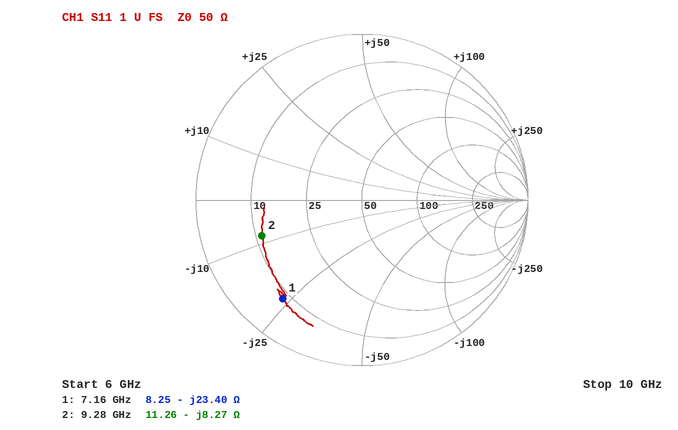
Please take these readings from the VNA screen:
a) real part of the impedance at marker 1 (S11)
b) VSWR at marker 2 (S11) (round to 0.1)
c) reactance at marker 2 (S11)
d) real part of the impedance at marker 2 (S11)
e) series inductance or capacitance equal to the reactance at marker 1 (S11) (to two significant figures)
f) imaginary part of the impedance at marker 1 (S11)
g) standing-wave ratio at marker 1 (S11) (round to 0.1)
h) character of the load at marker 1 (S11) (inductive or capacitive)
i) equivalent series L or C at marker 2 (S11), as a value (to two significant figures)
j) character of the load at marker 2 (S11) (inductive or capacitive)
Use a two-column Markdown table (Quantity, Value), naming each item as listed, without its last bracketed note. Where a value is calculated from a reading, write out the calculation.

| Quantity | Value |
|---|---|
| real part of the impedance at marker 1 | 8.25 Ω |
| VSWR at marker 2 (S11) | 4.6 |
| reactance at marker 2 | -8.27 Ω |
| real part of the impedance at marker 2 | 11.26 Ω |
| series inductance or capacitance equal to the reactance at marker 1 (S11) | C = 1/(2π × 7.16 GHz × 23.4 Ω) ≈ 950 fF |
| imaginary part of the impedance at marker 1 | -23.40 Ω |
| standing-wave ratio at marker 1 (S11) | 7.4 |
| character of the load at marker 1 (S11) | capacitive |
| equivalent series L or C at marker 2 (S11), as a value | C = 1/(2π × 9.28 GHz × 8.27 Ω) ≈ 2.1 pF |
| character of the load at marker 2 (S11) | capacitive |
